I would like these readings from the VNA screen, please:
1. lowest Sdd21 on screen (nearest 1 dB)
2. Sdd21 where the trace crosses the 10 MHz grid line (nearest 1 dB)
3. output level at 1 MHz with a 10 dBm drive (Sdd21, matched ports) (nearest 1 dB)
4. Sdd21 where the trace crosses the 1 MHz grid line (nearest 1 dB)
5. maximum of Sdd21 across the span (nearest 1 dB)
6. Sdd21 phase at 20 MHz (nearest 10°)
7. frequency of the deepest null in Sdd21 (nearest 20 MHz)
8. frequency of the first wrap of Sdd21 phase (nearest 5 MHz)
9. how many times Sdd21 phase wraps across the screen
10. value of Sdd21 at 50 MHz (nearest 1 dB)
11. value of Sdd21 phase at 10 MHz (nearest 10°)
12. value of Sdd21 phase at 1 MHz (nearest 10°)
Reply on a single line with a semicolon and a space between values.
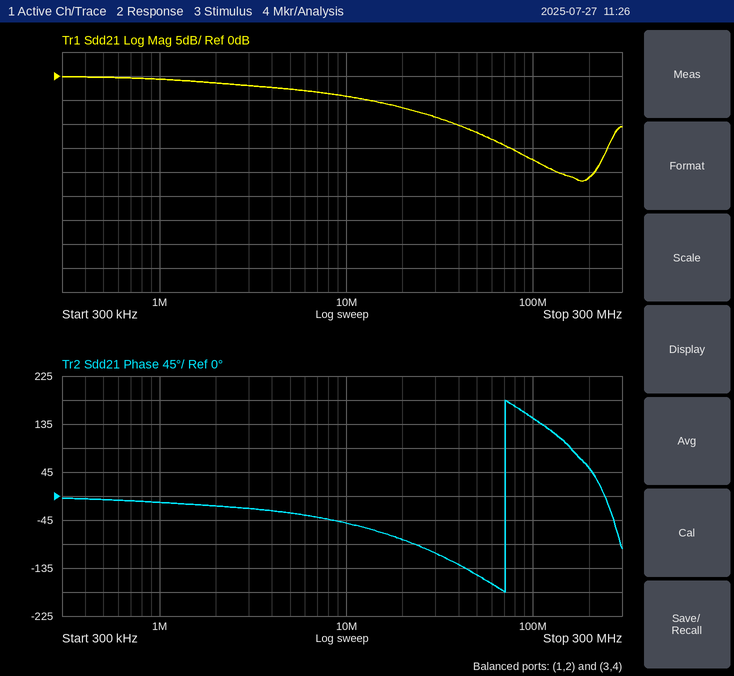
-22 dB; -4 dB; 9 dBm; -1 dB; 0 dB; -80°; 180 MHz; 70 MHz; 1; -12 dB; -50°; -10°
